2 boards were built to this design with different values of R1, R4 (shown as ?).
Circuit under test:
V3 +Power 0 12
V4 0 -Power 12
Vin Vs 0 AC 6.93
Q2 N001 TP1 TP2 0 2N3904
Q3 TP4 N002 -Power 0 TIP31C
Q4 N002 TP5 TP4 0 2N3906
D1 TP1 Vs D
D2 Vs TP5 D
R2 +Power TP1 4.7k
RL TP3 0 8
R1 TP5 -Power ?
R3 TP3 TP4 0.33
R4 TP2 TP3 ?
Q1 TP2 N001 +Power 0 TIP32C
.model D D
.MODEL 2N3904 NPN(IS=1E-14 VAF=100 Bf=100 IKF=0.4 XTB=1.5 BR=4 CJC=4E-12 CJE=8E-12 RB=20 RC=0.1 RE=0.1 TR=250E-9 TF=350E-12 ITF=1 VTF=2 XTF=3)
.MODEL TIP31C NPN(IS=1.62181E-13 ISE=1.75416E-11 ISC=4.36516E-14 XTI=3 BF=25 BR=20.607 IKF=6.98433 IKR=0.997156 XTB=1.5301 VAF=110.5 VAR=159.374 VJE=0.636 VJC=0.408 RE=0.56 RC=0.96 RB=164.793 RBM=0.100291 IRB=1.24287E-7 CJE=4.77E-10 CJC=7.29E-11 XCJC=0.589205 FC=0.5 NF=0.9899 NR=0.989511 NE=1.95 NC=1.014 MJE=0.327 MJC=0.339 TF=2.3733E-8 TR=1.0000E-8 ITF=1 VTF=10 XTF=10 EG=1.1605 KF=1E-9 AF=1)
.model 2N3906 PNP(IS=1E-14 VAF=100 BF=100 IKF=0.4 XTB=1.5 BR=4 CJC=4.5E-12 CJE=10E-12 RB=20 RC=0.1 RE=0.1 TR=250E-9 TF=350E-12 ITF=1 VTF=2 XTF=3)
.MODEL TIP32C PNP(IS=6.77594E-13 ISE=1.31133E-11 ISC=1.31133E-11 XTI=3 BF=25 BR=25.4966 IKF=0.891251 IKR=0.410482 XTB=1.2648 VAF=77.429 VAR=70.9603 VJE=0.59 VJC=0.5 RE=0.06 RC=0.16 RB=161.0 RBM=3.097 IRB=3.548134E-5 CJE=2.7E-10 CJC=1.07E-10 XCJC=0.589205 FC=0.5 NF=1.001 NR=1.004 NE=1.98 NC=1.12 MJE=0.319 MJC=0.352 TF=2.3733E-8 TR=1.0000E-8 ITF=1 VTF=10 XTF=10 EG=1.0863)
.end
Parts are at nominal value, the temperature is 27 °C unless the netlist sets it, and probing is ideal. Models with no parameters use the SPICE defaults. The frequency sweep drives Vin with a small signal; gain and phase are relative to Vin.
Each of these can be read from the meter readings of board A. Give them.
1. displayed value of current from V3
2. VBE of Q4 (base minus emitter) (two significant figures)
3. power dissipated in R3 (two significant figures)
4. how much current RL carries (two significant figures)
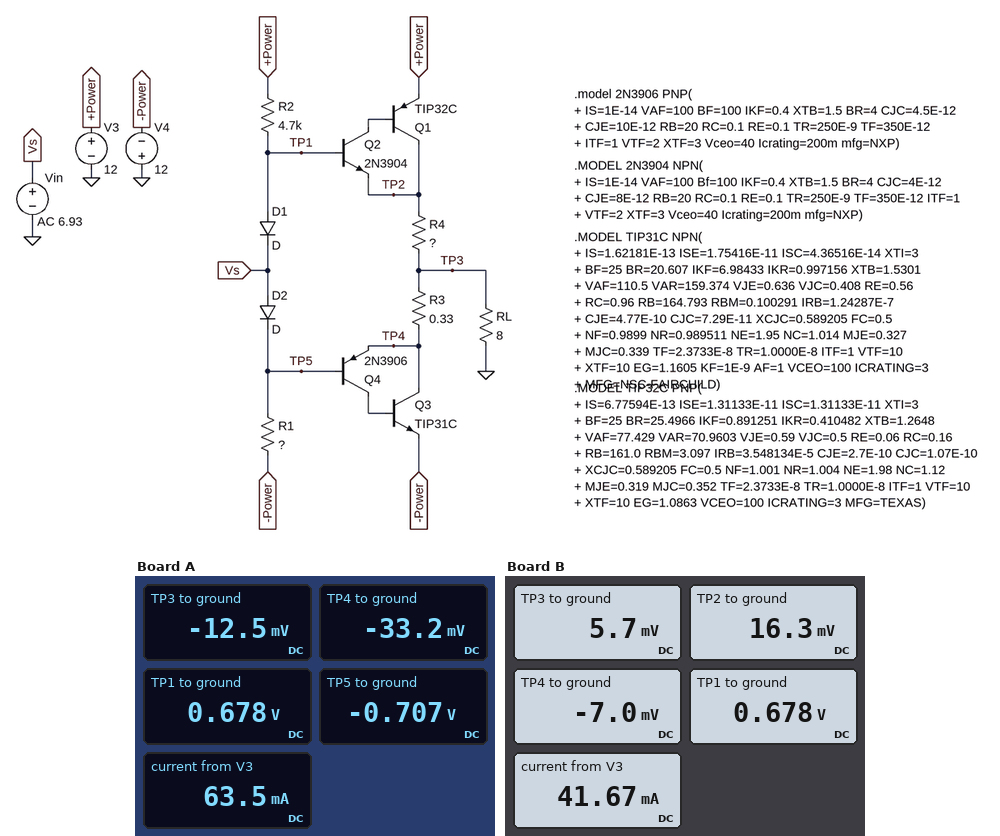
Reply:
63.5 mA
-670 mV
1.3 mW
1.6 mA
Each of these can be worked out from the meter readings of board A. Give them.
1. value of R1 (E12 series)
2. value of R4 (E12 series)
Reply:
1.5 kΩ
0.27 Ω
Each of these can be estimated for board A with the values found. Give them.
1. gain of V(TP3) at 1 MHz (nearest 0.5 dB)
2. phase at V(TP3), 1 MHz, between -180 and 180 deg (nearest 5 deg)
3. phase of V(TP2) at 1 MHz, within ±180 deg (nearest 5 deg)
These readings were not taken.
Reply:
-0.5 dB
-5 deg
-5 deg
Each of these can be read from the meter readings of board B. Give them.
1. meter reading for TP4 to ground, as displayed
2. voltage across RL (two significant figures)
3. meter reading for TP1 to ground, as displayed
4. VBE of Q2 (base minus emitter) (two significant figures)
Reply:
-7.0 mV
5.7 mV
0.678 V
660 mV
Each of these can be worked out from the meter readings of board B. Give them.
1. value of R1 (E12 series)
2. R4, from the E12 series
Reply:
6.8 kΩ
0.27 Ω
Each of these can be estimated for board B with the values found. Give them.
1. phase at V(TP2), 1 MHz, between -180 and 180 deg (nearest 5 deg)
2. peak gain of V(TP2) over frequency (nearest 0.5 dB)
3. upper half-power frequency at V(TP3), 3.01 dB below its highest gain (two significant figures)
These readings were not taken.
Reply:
-10 deg
-0.5 dB
4.4 MHz
